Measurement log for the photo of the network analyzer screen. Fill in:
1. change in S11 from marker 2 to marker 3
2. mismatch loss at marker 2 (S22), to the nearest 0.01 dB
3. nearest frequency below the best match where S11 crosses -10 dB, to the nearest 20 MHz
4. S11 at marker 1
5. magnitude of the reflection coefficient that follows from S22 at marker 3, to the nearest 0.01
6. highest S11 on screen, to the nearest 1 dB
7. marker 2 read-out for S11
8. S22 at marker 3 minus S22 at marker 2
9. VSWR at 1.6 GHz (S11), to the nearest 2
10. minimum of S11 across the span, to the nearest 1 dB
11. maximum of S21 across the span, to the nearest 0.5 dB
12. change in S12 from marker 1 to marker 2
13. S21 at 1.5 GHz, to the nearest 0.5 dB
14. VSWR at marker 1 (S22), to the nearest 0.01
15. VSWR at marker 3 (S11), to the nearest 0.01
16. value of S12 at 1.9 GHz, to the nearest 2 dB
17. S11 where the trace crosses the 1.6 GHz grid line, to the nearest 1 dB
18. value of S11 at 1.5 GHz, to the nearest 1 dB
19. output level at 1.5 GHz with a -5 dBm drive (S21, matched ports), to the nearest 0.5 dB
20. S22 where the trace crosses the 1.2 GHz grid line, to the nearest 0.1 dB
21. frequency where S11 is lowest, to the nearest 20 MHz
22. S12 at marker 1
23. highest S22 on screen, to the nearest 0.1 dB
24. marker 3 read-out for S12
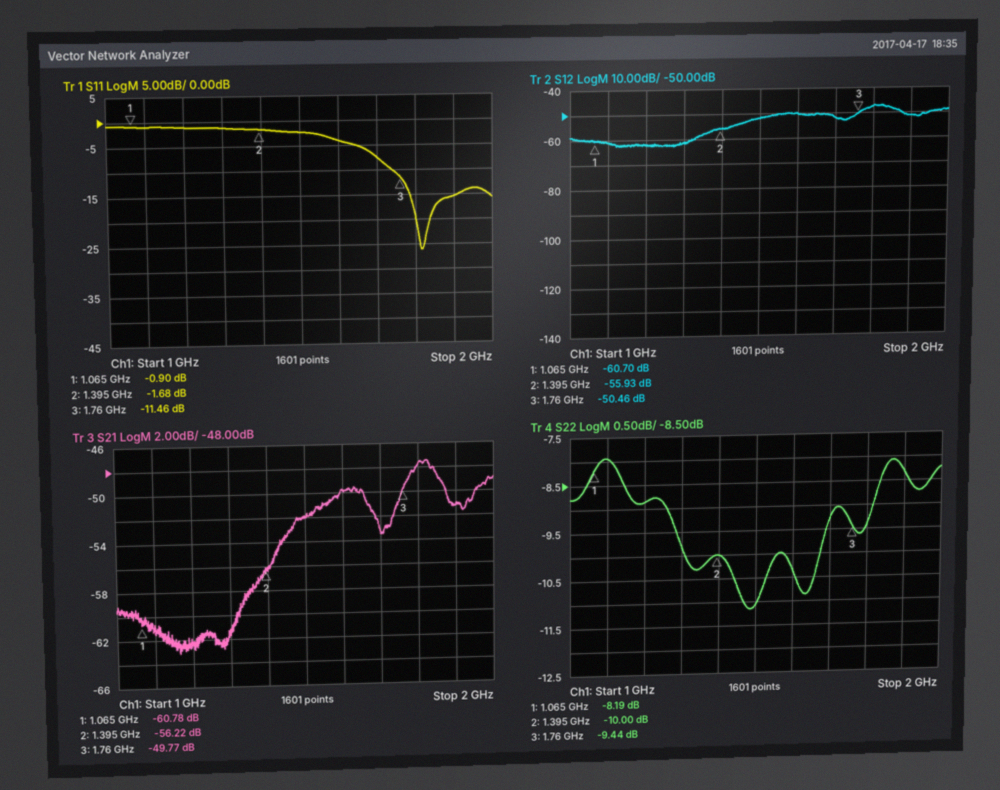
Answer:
-9.78 dB
0.46 dB
1.74 GHz
-0.90 dB
0.34
-1 dB
-1.68 dB
0.56 dB
4
-26 dB
-47.5 dB
4.77 dB
-52.0 dB
2.28
1.73
-52 dB
-4 dB
-2 dB
-57.0 dBm
-8.9 dB
1.82 GHz
-60.70 dB
-7.9 dB
-50.46 dB
